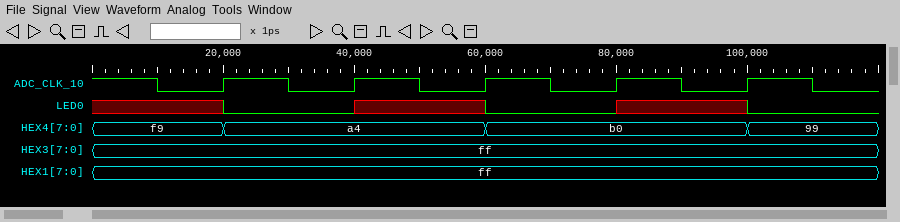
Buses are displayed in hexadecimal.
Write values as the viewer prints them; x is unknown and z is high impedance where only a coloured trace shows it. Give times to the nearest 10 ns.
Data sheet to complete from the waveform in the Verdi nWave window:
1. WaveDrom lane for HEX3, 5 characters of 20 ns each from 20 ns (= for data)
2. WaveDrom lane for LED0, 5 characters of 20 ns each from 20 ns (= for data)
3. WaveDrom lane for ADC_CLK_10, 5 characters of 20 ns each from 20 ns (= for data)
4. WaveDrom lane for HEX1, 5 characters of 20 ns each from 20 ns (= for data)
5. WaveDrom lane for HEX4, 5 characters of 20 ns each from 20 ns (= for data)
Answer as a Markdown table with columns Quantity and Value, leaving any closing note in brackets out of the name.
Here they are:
| Quantity | Value |
|---|---|
| WaveDrom lane for HEX3, 5 characters of 20 ns each from 20 ns | {name: 'HEX3', wave: '=....', data: 'ff'} |
| WaveDrom lane for LED0, 5 characters of 20 ns each from 20 ns | {name: 'LED0', wave: '0x0x0'} |
| WaveDrom lane for ADC_CLK_10, 5 characters of 20 ns each from 20 ns | {name: 'ADC_CLK_10', wave: 'p....'} |
| WaveDrom lane for HEX1, 5 characters of 20 ns each from 20 ns | {name: 'HEX1', wave: '=....', data: 'ff'} |
| WaveDrom lane for HEX4, 5 characters of 20 ns each from 20 ns | {name: 'HEX4', wave: '=.=.=', data: 'a4 b0 99'} |
